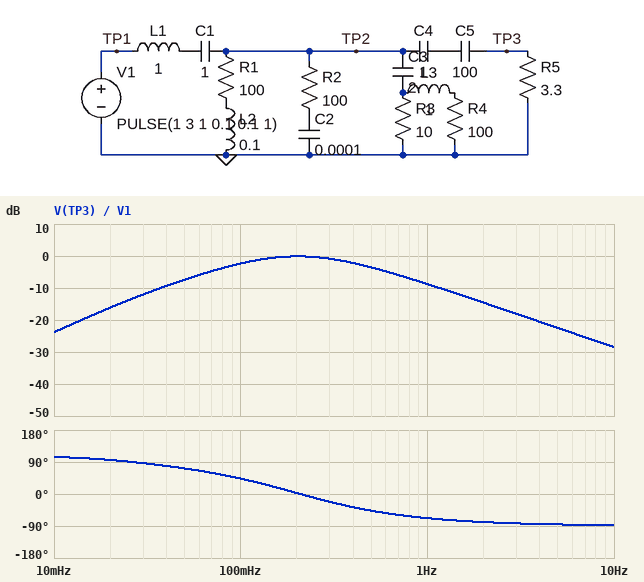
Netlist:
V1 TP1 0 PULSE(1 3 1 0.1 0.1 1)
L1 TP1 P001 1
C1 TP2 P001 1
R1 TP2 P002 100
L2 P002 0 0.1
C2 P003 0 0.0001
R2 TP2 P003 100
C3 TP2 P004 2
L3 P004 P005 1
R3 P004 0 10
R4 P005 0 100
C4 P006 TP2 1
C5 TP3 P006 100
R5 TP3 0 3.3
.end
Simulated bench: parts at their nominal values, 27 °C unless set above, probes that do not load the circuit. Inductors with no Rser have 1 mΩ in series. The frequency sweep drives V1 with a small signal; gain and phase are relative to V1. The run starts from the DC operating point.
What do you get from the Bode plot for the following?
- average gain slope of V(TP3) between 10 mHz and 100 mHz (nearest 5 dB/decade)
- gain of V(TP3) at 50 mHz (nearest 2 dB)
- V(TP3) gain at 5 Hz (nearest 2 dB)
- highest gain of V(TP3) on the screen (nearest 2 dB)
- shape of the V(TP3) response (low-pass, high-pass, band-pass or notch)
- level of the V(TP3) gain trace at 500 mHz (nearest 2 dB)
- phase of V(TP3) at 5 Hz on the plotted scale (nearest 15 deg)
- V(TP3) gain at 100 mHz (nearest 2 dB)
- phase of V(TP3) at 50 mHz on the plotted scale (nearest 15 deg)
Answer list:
20 dB/decade
-8 dB
-22 dB
0 dB
band-pass
-4 dB
-90 deg
-2 dB
75 deg
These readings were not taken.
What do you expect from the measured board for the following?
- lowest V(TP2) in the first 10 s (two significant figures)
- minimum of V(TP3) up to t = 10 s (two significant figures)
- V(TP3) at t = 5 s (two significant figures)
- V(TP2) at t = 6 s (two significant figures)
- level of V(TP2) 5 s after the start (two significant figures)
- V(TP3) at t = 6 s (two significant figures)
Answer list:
-470 mV
-750 mV
-250 mV
-93 mV
-220 mV
-78 mV
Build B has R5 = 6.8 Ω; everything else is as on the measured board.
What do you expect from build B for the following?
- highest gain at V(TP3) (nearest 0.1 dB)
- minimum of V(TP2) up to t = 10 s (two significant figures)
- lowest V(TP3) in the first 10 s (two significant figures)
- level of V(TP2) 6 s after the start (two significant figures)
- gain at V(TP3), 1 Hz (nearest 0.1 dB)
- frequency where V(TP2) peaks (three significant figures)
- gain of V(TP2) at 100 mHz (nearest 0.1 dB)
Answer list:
0 dB
-390 mV
-590 mV
-150 mV
-5.6 dB
184 mHz
-0.6 dB
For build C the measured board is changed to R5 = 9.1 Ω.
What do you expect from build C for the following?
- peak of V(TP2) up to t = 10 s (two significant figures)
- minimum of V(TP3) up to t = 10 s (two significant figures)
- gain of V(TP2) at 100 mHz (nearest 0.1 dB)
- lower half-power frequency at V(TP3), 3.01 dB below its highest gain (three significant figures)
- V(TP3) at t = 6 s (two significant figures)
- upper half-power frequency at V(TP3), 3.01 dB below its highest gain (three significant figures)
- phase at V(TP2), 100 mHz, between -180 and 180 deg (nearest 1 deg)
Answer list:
1.8 V
-520 mV
-0.4 dB
48.1 mHz
-210 mV
741 mHz
12 deg
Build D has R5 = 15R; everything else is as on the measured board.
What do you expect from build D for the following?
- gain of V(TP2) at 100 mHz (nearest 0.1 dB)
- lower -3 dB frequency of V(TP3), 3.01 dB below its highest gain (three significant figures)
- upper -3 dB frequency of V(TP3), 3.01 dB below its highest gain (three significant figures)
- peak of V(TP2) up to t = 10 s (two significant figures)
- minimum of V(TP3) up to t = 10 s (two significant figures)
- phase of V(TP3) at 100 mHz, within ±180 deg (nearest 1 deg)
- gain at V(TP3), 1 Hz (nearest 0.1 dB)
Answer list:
-0.3 dB
37.7 mHz
890 mHz
1.8 V
-420 mV
16 deg
-3.6 dB
